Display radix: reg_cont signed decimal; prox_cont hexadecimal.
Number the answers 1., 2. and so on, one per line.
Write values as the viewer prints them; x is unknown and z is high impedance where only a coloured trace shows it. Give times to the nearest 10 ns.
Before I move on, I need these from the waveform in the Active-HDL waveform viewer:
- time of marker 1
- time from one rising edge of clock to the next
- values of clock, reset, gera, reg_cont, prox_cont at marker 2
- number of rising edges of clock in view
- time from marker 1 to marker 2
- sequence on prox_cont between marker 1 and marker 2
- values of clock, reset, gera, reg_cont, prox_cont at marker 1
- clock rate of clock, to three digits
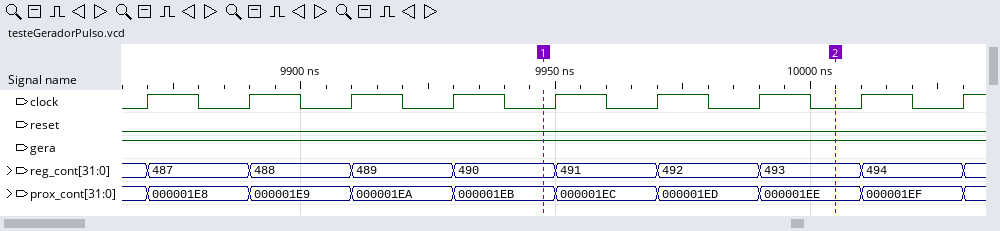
1. 9950 ns
2. 20 ns
3. clock=0, reset=0, gera=1, reg_cont=493, prox_cont=000001EE
4. 9
5. 60 ns
6. 000001EB, 000001EC, 000001ED, 000001EE
7. clock=0, reset=0, gera=1, reg_cont=490, prox_cont=000001EB
8. 50.0 MHz
